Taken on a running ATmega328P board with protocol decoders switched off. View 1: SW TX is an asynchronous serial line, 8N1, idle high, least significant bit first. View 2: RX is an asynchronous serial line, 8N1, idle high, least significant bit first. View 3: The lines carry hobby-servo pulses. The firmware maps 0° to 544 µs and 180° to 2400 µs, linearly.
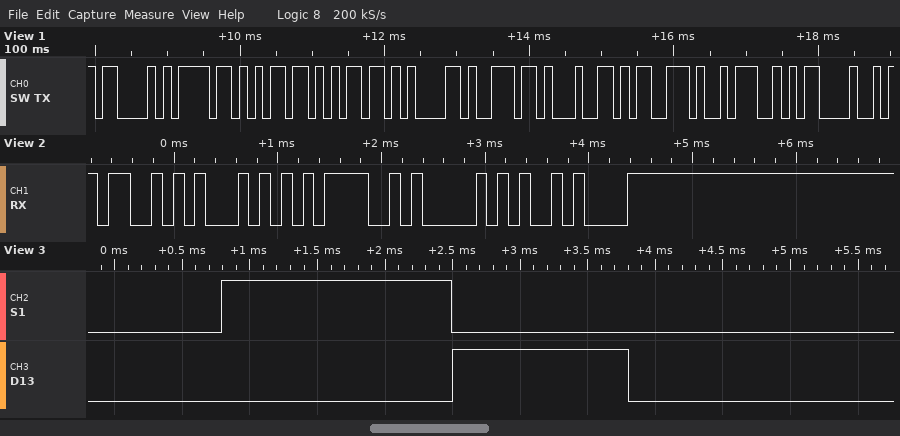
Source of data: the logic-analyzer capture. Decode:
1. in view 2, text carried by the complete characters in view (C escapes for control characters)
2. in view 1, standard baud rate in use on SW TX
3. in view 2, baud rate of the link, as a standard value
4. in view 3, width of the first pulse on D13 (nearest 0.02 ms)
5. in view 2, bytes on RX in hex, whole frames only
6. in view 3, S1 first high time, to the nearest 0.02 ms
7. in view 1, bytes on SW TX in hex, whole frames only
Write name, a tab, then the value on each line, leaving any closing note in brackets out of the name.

in view 2, text carried by the complete characters in view	"STOP\n"
in view 1, standard baud rate in use on SW TX	9600 baud
in view 2, baud rate of the link, as a standard value	9600 baud
in view 3, width of the first pulse on D13	1.30 ms
in view 2, bytes on RX in hex, whole frames only	53 54 4F 50 0A
in view 3, S1 first high time, to the nearest 0.02 ms	1.70 ms
in view 1, bytes on SW TX in hex, whole frames only	0x43 0x6F 0x6D 0x6D 0x61 0x6E 0x64 0x73 0x3A 0x0D
